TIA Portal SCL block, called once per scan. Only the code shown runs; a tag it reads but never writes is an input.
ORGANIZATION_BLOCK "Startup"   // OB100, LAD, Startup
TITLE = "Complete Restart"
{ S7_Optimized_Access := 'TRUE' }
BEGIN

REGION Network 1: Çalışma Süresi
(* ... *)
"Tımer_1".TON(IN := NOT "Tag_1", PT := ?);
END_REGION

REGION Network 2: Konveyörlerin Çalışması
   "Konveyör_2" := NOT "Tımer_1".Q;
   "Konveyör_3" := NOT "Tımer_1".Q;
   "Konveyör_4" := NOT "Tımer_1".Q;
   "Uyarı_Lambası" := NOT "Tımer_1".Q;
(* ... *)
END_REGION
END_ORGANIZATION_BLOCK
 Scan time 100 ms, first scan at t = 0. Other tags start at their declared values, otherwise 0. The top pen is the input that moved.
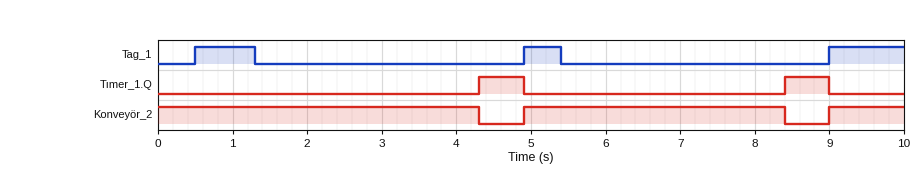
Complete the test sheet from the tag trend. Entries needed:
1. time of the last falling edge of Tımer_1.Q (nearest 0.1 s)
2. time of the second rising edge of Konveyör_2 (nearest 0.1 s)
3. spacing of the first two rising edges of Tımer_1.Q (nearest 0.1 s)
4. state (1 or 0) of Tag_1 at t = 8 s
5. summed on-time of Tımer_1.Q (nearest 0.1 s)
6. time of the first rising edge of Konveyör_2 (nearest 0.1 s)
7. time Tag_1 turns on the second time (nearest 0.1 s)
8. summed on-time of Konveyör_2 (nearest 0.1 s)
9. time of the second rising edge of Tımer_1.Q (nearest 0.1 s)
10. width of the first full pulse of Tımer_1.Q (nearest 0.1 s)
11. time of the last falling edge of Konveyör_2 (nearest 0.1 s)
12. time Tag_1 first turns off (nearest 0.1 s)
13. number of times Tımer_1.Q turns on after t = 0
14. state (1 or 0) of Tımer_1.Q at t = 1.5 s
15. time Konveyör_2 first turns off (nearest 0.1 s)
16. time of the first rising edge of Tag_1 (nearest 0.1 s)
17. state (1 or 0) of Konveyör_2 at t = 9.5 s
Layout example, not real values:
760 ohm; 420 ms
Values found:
9.0 s; 9.0 s; 4.1 s; 0; 1.2 s; 4.9 s; 4.9 s; 8.8 s; 8.4 s; 0.6 s; 8.4 s; 1.3 s; 2; 0; 4.3 s; 0.5 s; 1
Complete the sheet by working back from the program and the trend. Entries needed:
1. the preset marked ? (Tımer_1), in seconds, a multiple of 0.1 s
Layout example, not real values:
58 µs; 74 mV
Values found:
3.0 s
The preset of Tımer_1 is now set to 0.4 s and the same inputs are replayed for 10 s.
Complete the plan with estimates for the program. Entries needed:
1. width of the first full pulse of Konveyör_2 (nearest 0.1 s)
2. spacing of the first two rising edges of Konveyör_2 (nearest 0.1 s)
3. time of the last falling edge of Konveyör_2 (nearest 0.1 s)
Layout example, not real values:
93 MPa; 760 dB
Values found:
1.2 s; 4.4 s; 5.8 s
